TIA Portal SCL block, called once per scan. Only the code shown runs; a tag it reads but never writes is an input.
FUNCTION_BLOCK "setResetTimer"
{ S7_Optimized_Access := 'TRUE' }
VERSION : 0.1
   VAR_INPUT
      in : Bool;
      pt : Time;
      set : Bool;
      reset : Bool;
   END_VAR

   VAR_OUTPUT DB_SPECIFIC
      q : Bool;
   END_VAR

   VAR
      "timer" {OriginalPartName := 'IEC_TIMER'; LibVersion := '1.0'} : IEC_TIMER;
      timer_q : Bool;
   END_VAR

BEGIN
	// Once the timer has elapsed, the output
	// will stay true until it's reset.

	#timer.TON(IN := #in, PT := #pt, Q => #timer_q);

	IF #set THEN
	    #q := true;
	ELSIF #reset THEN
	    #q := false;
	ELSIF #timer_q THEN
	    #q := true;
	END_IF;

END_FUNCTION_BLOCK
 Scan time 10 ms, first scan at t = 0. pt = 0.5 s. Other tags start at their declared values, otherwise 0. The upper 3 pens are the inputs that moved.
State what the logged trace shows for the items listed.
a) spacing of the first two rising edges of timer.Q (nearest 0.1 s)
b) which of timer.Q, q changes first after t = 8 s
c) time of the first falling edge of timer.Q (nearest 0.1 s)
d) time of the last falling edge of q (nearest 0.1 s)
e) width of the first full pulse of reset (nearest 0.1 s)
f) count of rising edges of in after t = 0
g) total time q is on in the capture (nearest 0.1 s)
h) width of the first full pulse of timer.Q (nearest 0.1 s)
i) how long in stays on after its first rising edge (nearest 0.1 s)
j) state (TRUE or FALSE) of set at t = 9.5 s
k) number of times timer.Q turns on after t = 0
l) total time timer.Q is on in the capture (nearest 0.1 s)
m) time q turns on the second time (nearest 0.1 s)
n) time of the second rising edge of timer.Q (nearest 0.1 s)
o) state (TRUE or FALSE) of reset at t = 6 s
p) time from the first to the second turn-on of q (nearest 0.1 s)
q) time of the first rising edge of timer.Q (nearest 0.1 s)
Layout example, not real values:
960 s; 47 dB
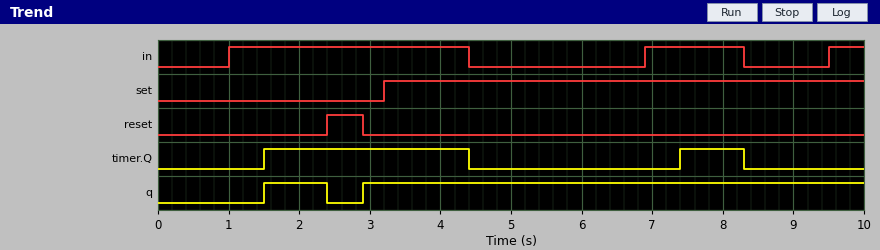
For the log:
5.9 s; timer.Q; 4.4 s; 2.4 s; 0.5 s; 3; 8.0 s; 2.9 s; 3.4 s; TRUE; 2; 3.8 s; 2.9 s; 7.4 s; FALSE; 1.4 s; 1.5 s
